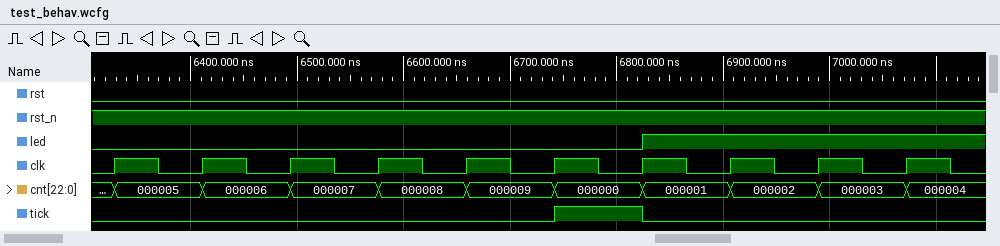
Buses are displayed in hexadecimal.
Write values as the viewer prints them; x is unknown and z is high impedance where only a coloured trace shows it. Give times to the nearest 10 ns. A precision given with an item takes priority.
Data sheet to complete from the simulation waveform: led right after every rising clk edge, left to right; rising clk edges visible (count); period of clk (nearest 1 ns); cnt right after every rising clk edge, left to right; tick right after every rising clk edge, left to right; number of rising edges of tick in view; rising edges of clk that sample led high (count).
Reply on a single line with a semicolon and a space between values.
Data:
0 0 0 0 0 0 1 1 1 1; 10; 83 ns; 000005, 000006, 000007, 000008, 000009, 000000, 000001, 000002, 000003, 000004; 0 0 0 0 0 1 0 0 0 0; 1; 3
